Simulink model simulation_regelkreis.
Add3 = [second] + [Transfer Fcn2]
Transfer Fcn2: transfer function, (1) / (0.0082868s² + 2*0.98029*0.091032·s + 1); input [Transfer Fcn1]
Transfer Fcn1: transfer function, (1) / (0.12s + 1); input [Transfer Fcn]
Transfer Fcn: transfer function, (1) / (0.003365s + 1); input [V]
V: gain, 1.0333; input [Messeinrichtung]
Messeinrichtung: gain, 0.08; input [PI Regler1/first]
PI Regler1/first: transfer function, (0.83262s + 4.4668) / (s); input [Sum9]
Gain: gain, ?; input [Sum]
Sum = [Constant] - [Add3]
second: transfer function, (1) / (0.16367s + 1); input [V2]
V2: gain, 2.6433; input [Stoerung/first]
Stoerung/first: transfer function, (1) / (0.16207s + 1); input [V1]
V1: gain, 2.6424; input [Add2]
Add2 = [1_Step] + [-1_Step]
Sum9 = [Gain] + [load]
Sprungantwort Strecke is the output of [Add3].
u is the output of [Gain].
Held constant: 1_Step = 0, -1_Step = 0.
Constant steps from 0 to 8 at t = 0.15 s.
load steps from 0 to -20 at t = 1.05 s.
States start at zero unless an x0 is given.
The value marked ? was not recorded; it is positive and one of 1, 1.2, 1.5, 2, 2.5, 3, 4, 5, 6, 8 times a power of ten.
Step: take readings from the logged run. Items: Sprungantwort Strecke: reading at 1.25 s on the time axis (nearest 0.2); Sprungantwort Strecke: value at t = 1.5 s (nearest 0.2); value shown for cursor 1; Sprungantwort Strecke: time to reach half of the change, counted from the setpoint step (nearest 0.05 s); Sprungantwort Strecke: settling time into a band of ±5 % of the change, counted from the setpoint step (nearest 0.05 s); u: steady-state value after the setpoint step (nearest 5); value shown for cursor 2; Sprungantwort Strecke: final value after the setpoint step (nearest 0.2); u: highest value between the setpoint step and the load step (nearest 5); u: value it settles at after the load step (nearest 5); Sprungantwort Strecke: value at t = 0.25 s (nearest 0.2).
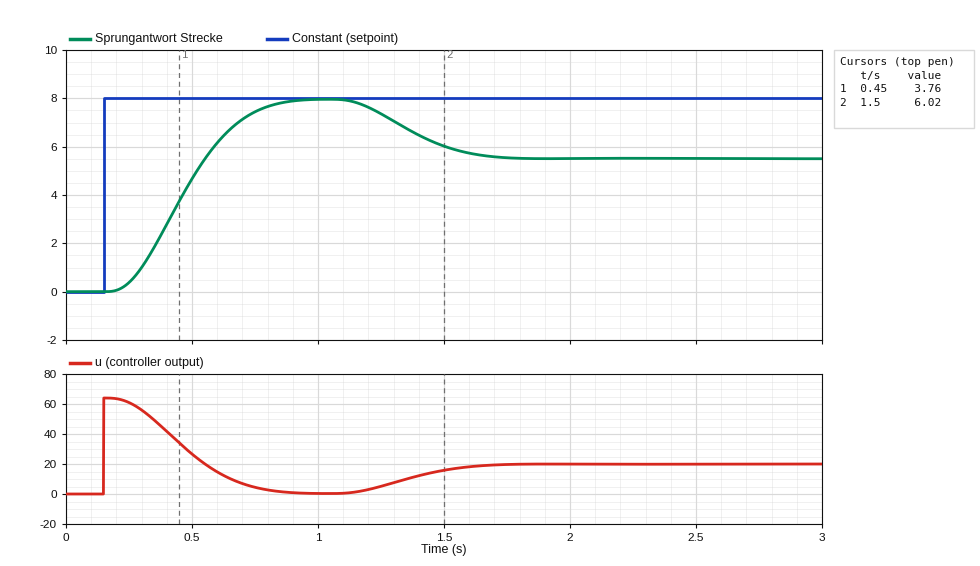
7.4
6.0
3.76
0.30 s
0.65 s
0
6.02
8.0
65
20
0.4
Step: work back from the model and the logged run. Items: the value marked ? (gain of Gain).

8
